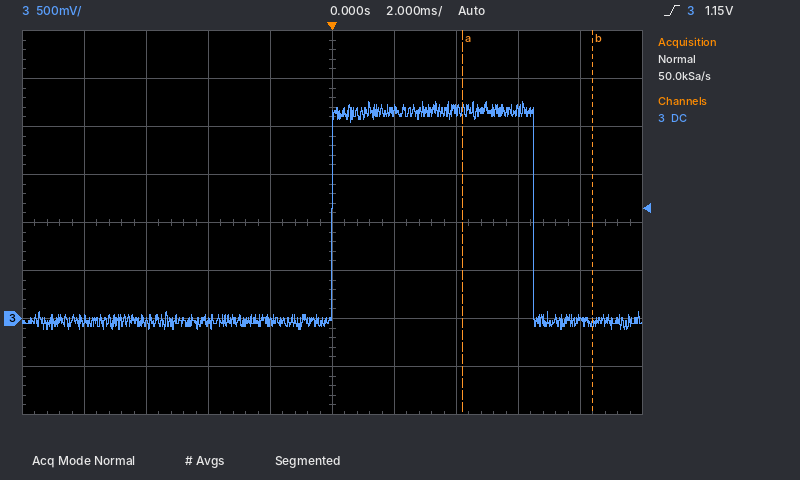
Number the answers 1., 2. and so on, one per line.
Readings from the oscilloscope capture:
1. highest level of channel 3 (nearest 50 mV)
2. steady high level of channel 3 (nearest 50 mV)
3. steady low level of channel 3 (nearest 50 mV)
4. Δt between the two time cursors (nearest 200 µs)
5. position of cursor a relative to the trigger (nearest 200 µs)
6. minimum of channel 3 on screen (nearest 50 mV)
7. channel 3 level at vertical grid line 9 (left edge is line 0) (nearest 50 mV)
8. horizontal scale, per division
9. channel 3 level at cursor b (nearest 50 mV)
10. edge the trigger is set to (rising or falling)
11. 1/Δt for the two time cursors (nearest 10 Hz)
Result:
1. 2.25 V
2. 2.15 V
3. -50 mV
4. 4.2 ms
5. +4.2 ms
6. -100 mV
7. 0 mV
8. 2 ms
9. -50 mV
10. rising
11. 240 Hz
